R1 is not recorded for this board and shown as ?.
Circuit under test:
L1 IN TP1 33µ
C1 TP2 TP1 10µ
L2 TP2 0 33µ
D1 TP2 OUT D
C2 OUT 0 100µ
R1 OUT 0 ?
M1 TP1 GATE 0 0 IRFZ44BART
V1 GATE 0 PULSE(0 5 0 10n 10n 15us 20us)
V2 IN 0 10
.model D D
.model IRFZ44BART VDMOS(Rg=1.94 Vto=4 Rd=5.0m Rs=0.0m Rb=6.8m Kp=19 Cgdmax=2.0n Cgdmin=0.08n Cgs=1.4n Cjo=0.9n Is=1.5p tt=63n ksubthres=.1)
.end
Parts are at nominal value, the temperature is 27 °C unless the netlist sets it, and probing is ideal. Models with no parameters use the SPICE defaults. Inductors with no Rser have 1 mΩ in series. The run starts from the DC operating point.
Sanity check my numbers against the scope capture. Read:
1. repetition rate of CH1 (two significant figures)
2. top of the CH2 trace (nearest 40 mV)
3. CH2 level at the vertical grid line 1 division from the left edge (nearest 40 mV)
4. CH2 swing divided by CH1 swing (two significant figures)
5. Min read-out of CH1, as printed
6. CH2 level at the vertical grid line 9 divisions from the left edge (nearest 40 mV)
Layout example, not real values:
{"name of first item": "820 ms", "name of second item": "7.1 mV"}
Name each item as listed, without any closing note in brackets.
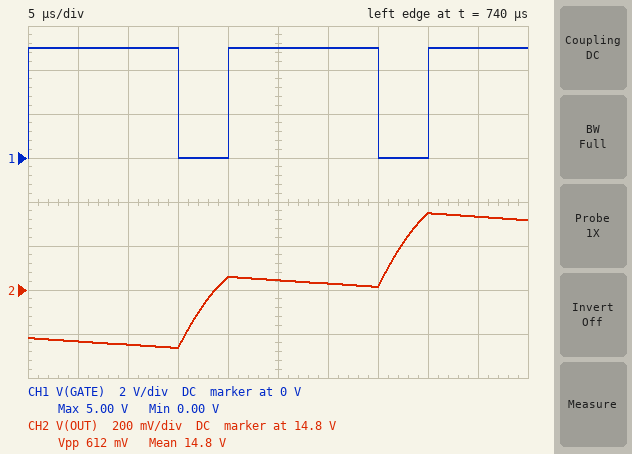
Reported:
{"repetition rate of CH1": "50 kHz", "top of the CH2 trace": "15.16 V", "CH2 level at the vertical grid line 1 division from the left edge": "14.56 V", "CH2 swing divided by CH1 swing": "0.12", "Min read-out of CH1, as printed": "0.00 V", "CH2 level at the vertical grid line 9 divisions from the left edge": "15.12 V"}
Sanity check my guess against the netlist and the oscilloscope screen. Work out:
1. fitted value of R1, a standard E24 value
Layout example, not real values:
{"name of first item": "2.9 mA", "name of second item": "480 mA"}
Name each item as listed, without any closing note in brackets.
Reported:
{"fitted value of R1, a standard E24 value": "47 Ω"}
